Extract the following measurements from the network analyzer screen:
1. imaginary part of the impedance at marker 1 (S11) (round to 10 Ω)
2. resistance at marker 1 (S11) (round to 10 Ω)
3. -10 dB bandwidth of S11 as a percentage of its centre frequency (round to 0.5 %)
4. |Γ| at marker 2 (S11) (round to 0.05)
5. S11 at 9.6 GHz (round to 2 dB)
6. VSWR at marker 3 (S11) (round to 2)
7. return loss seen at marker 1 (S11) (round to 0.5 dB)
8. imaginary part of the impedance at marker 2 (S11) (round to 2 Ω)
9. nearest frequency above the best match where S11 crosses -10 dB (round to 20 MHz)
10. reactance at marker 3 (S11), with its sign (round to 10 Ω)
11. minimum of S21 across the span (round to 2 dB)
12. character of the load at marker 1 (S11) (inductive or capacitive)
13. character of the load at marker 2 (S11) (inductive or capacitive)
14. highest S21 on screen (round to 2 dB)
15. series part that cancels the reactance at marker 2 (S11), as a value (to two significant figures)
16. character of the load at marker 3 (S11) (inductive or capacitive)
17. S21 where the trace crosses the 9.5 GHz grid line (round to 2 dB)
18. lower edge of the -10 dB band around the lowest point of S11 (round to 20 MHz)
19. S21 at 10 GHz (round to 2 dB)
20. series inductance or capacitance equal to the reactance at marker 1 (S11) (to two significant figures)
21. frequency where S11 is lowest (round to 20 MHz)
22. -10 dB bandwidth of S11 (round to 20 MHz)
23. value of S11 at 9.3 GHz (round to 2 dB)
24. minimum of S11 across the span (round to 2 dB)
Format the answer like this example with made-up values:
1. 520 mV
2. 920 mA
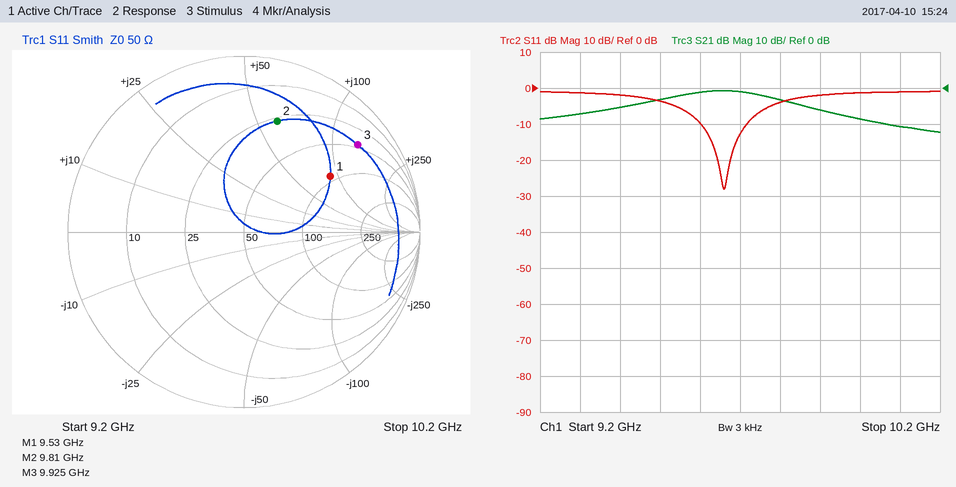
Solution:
1. +90 Ω
2. 90 Ω
3. 1.0 %
4. 0.65
5. -10 dB
6. 10
7. 4.5 dB
8. +60 Ω
9. 9.72 GHz
10. +130 Ω
11. -12 dB
12. inductive
13. inductive
14. 0 dB
15. 270 fF
16. inductive
17. -4 dB
18. 9.60 GHz
19. -8 dB
20. 1.5 nH
21. 9.66 GHz
22. 120 MHz
23. -2 dB
24. -28 dB
